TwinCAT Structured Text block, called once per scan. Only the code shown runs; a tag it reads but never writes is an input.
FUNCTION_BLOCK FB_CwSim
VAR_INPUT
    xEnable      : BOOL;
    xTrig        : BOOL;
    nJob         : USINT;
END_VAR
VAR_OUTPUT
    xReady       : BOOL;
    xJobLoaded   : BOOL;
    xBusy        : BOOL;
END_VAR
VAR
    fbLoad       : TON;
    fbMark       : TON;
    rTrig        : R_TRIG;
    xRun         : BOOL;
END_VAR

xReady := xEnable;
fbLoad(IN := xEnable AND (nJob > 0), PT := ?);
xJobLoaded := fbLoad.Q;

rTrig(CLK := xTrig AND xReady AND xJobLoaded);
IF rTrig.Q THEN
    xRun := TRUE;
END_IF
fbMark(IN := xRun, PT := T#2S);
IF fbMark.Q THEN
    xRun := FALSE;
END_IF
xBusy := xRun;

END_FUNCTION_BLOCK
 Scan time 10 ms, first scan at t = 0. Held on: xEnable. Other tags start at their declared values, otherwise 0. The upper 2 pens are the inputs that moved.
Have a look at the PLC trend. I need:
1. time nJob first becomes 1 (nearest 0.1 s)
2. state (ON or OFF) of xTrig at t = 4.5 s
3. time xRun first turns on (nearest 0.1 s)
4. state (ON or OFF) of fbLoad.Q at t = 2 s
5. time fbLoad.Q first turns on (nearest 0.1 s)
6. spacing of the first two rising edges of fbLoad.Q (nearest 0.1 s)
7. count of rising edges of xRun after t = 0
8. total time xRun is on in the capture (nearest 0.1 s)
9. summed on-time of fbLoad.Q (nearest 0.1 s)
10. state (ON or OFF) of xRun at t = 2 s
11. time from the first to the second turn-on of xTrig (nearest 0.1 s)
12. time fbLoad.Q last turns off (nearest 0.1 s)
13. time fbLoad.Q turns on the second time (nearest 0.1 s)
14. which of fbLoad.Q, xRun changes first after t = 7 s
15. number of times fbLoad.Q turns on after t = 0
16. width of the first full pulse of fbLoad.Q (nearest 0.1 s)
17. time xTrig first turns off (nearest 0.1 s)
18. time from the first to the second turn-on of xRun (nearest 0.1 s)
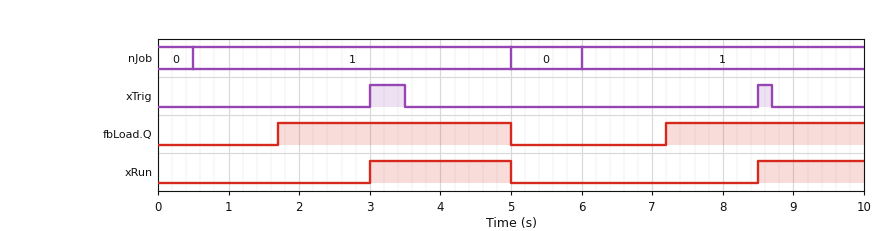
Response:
0.5 s
OFF
3.0 s
ON
1.7 s
5.5 s
2
3.5 s
6.1 s
OFF
5.5 s
5.0 s
7.2 s
fbLoad.Q
2
3.3 s
3.5 s
5.5 s
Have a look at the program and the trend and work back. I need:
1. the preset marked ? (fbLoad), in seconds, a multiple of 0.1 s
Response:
1.2 s
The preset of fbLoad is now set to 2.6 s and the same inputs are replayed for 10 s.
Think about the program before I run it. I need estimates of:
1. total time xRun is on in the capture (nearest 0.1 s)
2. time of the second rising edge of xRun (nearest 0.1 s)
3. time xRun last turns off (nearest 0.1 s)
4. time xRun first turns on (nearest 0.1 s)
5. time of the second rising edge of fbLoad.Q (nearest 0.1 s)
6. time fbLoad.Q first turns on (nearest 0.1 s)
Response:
3.4 s
8.6 s
5.1 s
3.1 s
8.6 s
3.1 s
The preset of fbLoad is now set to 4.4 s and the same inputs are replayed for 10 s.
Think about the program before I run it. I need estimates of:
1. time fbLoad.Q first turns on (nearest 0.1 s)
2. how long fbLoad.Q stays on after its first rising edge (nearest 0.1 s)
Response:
4.9 s
0.1 s
